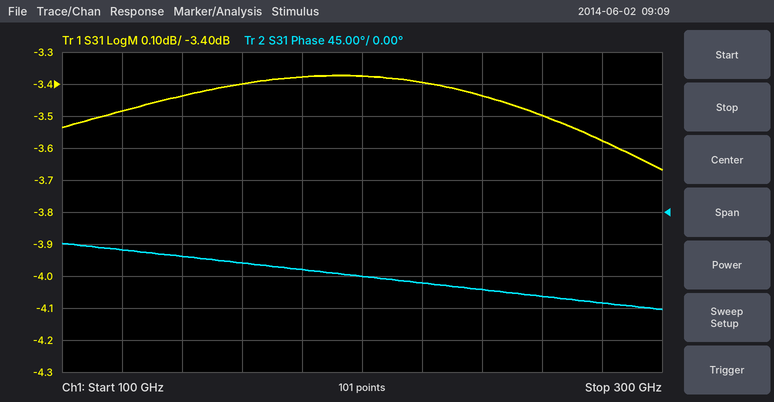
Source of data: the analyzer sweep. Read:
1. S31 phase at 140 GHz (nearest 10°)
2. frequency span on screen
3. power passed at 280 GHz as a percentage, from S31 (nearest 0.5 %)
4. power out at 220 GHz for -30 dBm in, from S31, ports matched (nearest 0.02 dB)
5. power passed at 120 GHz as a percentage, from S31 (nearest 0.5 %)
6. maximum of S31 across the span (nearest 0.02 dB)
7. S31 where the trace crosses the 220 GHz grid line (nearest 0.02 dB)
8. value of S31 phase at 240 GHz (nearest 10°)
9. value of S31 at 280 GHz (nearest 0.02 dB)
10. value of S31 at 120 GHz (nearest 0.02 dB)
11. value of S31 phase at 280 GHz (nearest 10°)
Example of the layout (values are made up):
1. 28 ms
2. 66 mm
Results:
1. -60°
2. 200 GHz
3. 44.0 %
4. -33.40 dBm
5. 45.0 %
6. -3.38 dB
7. -3.40 dB
8. -110°
9. -3.58 dB
10. -3.48 dB
11. -130°
